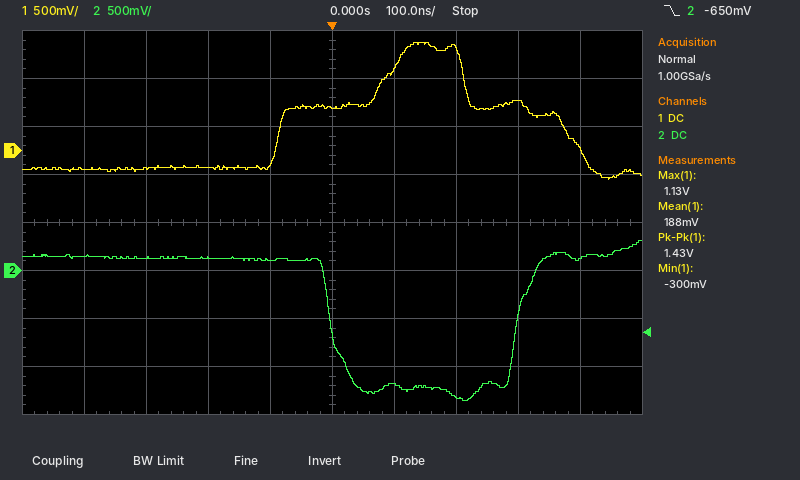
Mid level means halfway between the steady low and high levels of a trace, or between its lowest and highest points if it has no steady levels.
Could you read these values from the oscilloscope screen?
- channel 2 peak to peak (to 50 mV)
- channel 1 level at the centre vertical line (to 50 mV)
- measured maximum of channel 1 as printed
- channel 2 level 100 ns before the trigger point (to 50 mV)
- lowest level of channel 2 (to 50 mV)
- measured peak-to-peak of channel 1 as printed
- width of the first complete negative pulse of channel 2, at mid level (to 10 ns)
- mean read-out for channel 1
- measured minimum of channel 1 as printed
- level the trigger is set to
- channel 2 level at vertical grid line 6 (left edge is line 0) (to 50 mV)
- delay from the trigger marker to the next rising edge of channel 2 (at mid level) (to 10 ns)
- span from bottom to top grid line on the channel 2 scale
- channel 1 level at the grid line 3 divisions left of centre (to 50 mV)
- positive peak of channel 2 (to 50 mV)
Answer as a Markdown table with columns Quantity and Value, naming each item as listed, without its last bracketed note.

| Quantity | Value |
|---|---|
| channel 2 peak to peak | 1.65 V |
| channel 1 level at the centre vertical line | 450 mV |
| measured maximum of channel 1 as printed | 1.13 V |
| channel 2 level 100 ns before the trigger point | 100 mV |
| lowest level of channel 2 | -1.35 V |
| measured peak-to-peak of channel 1 as printed | 1.43 V |
| width of the first complete negative pulse of channel 2, at mid level | 300 ns |
| mean read-out for channel 1 | 188 mV |
| measured minimum of channel 1 as printed | -300 mV |
| level the trigger is set to | -650 mV |
| channel 2 level at vertical grid line 6 (left edge is line 0) | -1.20 V |
| delay from the trigger marker to the next rising edge of channel 2 (at mid level) | 300 ns |
| span from bottom to top grid line on the channel 2 scale | 4 V |
| channel 1 level at the grid line 3 divisions left of centre | -200 mV |
| positive peak of channel 2 | 300 mV |
